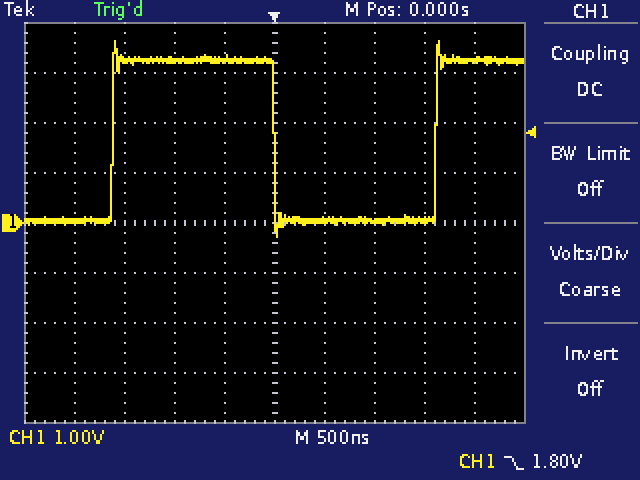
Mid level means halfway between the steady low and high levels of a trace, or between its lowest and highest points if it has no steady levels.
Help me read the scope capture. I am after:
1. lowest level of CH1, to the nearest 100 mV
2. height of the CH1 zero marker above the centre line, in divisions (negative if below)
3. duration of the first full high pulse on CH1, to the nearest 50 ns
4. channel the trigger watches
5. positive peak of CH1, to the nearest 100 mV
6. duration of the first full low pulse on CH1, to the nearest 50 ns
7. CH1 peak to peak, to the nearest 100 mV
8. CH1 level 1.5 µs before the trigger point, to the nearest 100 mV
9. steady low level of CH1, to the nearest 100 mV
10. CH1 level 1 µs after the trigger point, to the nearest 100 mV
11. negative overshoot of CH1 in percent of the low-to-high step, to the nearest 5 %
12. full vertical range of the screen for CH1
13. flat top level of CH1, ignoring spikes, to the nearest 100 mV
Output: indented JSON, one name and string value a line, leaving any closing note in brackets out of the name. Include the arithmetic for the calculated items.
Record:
{
  "lowest level of CH1, to the nearest 100 mV": "-300 mV",
  "height of the CH1 zero marker above the centre line, in divisions": "0.0 div",
  "duration of the first full high pulse on CH1, to the nearest 50 ns": "1.60 µs",
  "channel the trigger watches": "CH1",
  "positive peak of CH1, to the nearest 100 mV": "3.6 V",
  "duration of the first full low pulse on CH1, to the nearest 50 ns": "1.60 µs",
  "CH1 peak to peak, to the nearest 100 mV": "3.6 V − (-300 mV) = 3.9 V",
  "CH1 level 1.5 µs before the trigger point, to the nearest 100 mV": "3.3 V",
  "steady low level of CH1, to the nearest 100 mV": "0.0 V",
  "CH1 level 1 µs after the trigger point, to the nearest 100 mV": "0.0 V",
  "negative overshoot of CH1 in percent of the low-to-high step, to the nearest 5 %": "10 %",
  "full vertical range of the screen for CH1": "8 V",
  "flat top level of CH1, ignoring spikes, to the nearest 100 mV": "3.2 V"
}
